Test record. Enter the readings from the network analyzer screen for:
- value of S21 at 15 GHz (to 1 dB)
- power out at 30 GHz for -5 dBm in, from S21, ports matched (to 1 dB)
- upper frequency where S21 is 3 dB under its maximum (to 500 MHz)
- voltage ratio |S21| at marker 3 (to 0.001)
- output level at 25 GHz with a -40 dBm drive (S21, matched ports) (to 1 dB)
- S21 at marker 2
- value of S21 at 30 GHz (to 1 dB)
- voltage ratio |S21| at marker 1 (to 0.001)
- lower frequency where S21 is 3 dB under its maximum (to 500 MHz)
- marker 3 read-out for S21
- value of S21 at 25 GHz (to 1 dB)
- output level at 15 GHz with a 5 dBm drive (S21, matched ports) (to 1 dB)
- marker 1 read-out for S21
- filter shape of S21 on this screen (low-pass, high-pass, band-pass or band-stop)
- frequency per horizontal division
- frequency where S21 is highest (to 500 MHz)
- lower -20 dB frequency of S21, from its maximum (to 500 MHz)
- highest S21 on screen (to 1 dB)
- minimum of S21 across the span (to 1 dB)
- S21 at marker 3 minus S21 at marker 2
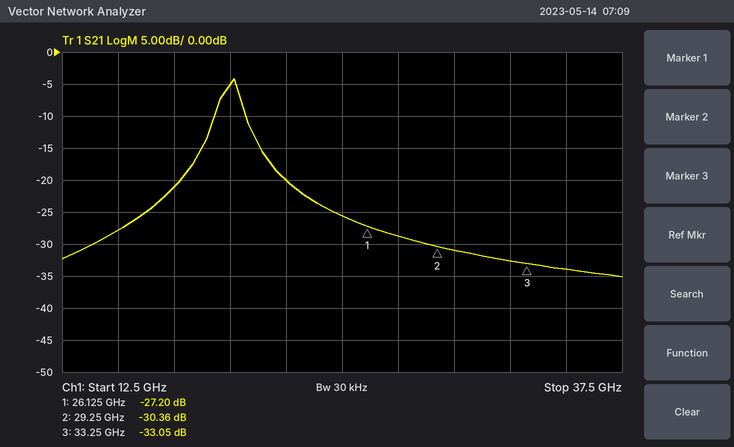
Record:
-28 dB
-36 dBm
20.5 GHz
0.022
-66 dBm
-30.36 dB
-31 dB
0.044
19.5 GHz
-33.05 dB
-26 dB
-23 dBm
-27.20 dB
band-pass
2.5 GHz
20.0 GHz
16.5 GHz
-4 dB
-35 dB
-2.69 dB
